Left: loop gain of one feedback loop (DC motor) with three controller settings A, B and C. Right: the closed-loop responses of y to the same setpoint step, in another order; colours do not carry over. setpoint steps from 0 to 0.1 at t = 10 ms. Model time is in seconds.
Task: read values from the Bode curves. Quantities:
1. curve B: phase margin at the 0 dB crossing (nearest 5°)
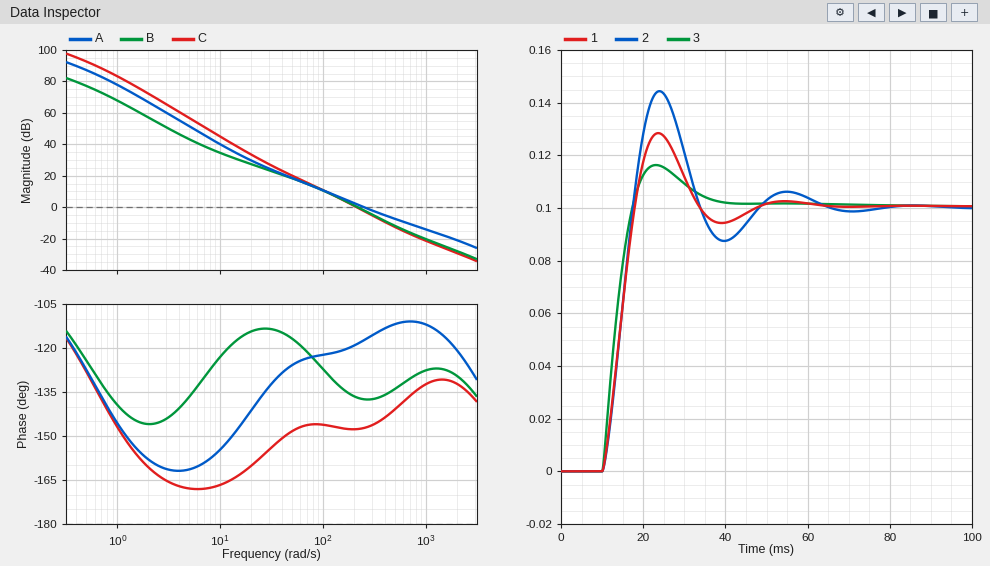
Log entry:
45°
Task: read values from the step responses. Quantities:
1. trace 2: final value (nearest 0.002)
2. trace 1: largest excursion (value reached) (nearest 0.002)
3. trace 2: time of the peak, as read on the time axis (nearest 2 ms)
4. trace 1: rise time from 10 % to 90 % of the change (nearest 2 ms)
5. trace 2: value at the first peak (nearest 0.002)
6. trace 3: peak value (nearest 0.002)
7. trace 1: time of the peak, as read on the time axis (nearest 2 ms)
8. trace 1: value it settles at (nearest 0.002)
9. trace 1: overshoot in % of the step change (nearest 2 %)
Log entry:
0.100
0.128
24 ms
6 ms
0.144
0.116
24 ms
0.100
28 %
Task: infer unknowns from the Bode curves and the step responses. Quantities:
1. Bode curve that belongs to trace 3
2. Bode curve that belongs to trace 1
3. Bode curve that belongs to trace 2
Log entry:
A
B
C
